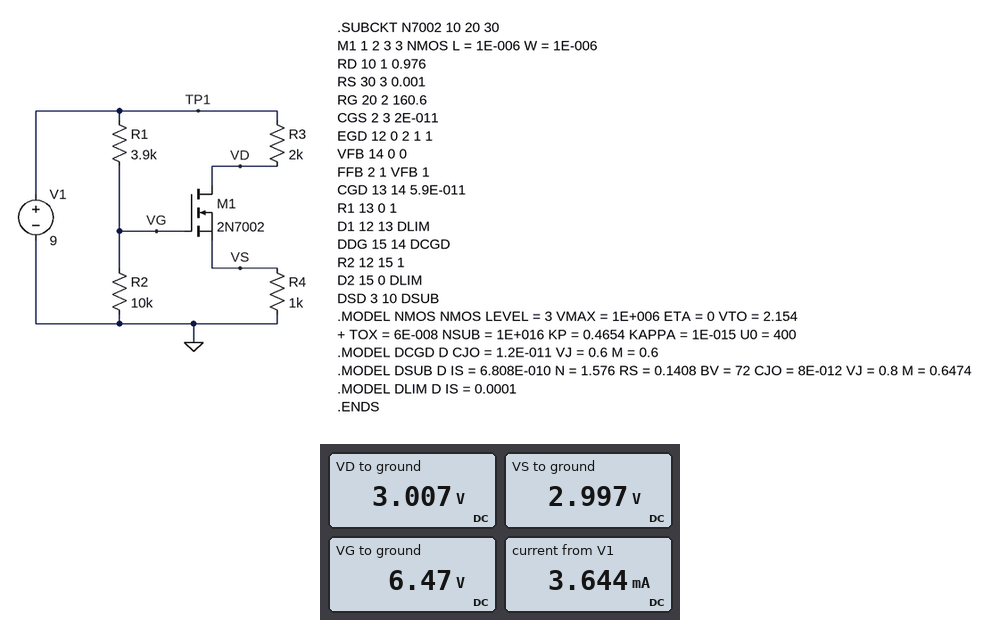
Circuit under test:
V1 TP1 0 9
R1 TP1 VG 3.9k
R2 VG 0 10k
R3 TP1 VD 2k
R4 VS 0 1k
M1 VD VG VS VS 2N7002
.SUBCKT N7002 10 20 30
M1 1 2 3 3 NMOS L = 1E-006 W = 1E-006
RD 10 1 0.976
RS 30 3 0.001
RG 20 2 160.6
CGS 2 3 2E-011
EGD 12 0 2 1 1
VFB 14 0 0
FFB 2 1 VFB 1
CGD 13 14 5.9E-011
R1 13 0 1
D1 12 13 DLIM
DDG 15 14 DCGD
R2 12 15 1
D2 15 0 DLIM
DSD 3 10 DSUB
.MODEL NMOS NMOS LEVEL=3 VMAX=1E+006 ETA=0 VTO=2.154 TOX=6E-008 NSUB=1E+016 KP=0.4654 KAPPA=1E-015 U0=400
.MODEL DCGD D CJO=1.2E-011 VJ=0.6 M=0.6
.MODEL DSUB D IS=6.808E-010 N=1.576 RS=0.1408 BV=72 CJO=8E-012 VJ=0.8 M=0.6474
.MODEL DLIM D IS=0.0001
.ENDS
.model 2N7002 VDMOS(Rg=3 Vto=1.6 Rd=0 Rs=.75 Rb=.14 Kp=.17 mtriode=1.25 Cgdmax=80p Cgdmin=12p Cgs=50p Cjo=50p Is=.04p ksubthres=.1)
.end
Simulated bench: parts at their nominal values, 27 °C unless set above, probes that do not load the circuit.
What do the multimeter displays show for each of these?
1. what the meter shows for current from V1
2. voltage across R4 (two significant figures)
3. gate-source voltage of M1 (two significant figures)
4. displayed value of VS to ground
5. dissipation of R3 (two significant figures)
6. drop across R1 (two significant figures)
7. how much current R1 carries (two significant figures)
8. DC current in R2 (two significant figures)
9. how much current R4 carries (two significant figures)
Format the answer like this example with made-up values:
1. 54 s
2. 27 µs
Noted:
1. 3.644 mA
2. 3.0 V
3. 3.5 V
4. 2.997 V
5. 18 mW
6. 2.5 V
7. 650 µA
8. 650 µA
9. 3.0 mA
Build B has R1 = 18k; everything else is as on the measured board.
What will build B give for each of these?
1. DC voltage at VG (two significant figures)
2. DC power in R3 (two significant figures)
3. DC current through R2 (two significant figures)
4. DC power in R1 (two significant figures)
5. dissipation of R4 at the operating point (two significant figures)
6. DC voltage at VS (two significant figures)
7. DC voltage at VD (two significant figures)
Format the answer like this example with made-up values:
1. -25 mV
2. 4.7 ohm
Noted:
1. 3.2 V
2. 4.6 mW
3. 320 µA
4. 1.9 mW
5. 2.3 mW
6. 1.5 V
7. 6.0 V
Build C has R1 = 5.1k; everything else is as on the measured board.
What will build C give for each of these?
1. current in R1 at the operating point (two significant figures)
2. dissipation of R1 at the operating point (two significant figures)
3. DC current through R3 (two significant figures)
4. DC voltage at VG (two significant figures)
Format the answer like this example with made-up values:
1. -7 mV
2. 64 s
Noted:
1. 600 µA
2. 1.8 mW
3. 3.0 mA
4. 6.0 V
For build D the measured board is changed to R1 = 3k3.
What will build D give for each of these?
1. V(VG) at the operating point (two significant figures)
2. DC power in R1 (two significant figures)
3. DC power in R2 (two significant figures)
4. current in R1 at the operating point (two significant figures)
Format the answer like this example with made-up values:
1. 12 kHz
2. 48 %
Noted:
1. 6.8 V
2. 1.5 mW
3. 4.6 mW
4. 680 µA
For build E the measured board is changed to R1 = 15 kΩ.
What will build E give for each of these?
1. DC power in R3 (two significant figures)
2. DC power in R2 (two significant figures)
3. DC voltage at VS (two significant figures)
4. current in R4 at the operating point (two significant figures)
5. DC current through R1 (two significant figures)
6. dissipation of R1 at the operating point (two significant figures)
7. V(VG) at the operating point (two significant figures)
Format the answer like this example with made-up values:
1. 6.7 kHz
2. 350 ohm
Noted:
1. 7.0 mW
2. 1.3 mW
3. 1.9 V
4. 1.9 mA
5. 360 µA
6. 1.9 mW
7. 3.6 V
